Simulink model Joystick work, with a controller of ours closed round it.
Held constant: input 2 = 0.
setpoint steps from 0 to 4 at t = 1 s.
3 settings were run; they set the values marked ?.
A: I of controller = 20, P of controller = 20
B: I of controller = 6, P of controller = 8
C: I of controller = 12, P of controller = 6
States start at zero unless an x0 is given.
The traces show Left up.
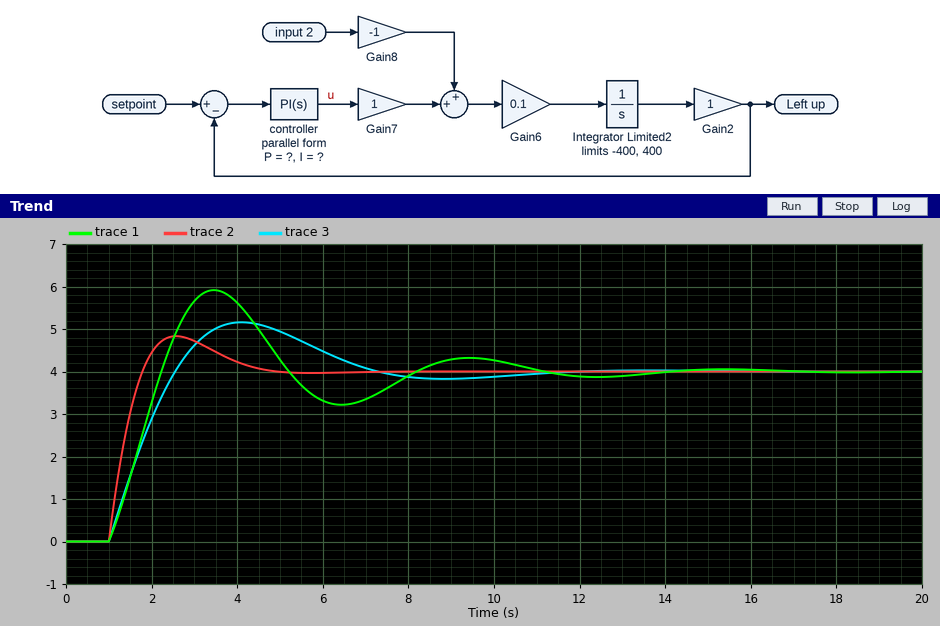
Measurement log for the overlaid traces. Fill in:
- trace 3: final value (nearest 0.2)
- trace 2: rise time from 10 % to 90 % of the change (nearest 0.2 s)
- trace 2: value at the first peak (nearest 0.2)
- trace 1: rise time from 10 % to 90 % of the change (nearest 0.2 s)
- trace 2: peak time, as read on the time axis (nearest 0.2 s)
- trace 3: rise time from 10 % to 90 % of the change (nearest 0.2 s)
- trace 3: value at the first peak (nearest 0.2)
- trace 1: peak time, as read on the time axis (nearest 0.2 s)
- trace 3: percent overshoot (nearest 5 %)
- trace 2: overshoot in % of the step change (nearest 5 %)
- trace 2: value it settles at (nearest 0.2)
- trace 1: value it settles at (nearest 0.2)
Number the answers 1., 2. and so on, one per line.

1. 4.0
2. 0.6 s
3. 4.8
4. 1.0 s
5. 2.6 s
6. 1.2 s
7. 5.2
8. 3.4 s
9. 30 %
10. 20 %
11. 4.0
12. 4.0
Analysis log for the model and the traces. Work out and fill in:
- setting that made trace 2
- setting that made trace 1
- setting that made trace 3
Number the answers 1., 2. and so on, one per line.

1. A
2. C
3. B
